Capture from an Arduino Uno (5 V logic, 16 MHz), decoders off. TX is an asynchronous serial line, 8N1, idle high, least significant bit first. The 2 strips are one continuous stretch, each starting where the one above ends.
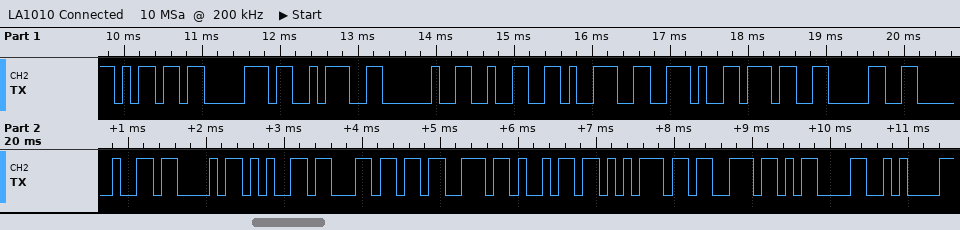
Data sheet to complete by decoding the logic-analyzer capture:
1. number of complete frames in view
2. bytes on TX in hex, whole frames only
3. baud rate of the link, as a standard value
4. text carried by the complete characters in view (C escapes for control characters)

19
6D 70 3A 20 32 39 2E 37 30 20 43 65 6C 73 69 75 73 0D 0A
9600 baud
"mp: 29.70 Celsius\r\n"
